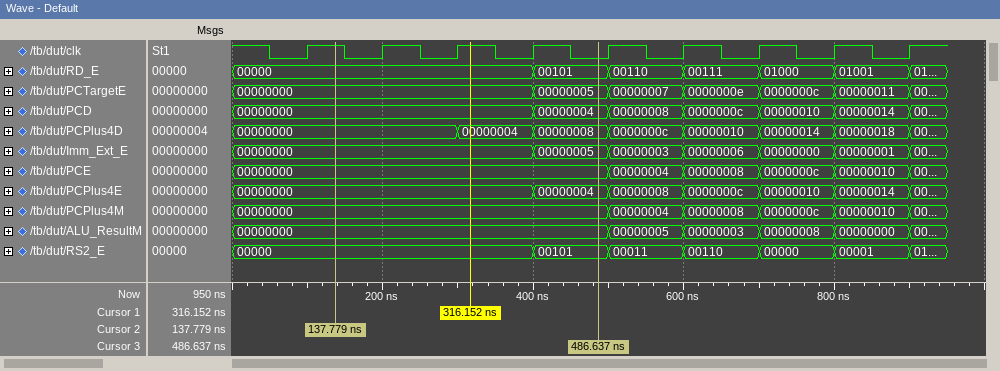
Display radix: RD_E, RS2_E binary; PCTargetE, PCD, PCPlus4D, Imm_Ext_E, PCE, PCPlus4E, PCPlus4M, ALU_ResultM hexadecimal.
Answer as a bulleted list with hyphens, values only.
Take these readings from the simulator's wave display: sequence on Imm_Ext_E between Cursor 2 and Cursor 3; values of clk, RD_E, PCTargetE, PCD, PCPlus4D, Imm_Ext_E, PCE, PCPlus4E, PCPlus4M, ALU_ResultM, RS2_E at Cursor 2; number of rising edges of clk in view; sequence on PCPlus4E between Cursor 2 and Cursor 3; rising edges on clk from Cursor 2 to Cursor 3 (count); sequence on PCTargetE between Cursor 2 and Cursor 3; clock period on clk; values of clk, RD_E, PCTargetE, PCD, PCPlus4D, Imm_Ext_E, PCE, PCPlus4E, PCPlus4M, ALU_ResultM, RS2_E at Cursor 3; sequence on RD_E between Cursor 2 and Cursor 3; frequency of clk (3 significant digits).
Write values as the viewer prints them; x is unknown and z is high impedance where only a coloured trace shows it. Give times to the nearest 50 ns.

- 00000000, 00000005
- clk=1, RD_E=00000, PCTargetE=00000000, PCD=00000000, PCPlus4D=00000000, Imm_Ext_E=00000000, PCE=00000000, PCPlus4E=00000000, PCPlus4M=00000000, ALU_ResultM=00000000, RS2_E=00000
- 9
- 00000000, 00000004
- 3
- 00000000, 00000005
- 100 ns
- clk=0, RD_E=00101, PCTargetE=00000005, PCD=00000004, PCPlus4D=00000008, Imm_Ext_E=00000005, PCE=00000000, PCPlus4E=00000004, PCPlus4M=00000000, ALU_ResultM=00000000, RS2_E=00101
- 00000, 00101
- 10.0 MHz
